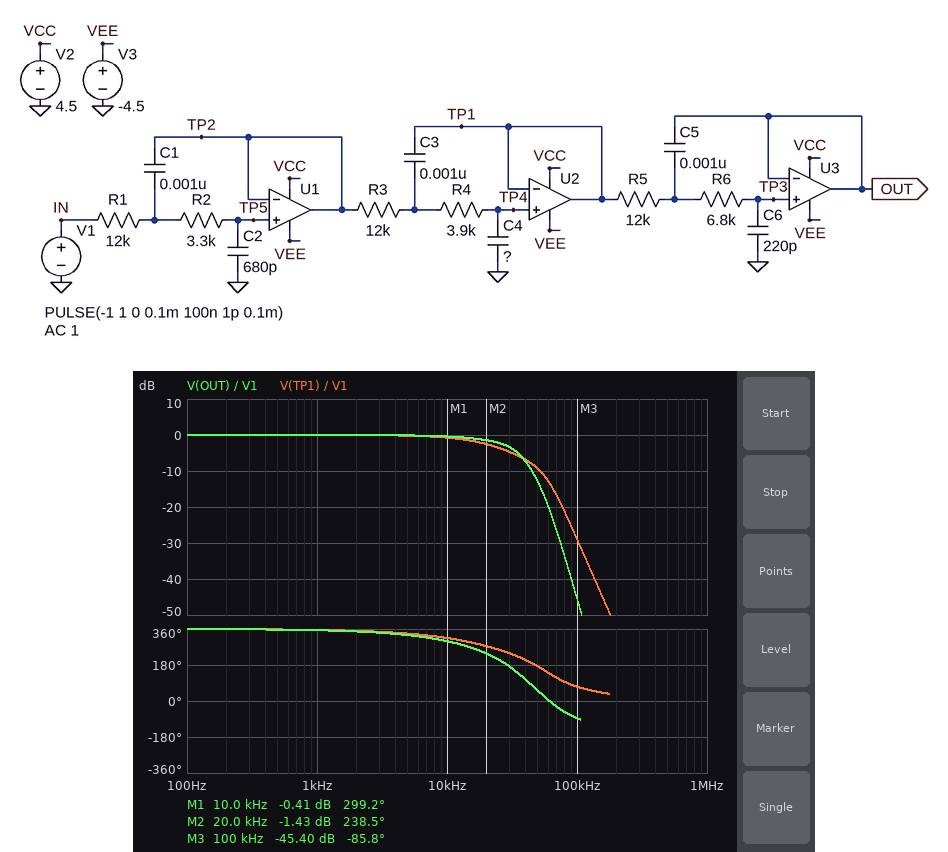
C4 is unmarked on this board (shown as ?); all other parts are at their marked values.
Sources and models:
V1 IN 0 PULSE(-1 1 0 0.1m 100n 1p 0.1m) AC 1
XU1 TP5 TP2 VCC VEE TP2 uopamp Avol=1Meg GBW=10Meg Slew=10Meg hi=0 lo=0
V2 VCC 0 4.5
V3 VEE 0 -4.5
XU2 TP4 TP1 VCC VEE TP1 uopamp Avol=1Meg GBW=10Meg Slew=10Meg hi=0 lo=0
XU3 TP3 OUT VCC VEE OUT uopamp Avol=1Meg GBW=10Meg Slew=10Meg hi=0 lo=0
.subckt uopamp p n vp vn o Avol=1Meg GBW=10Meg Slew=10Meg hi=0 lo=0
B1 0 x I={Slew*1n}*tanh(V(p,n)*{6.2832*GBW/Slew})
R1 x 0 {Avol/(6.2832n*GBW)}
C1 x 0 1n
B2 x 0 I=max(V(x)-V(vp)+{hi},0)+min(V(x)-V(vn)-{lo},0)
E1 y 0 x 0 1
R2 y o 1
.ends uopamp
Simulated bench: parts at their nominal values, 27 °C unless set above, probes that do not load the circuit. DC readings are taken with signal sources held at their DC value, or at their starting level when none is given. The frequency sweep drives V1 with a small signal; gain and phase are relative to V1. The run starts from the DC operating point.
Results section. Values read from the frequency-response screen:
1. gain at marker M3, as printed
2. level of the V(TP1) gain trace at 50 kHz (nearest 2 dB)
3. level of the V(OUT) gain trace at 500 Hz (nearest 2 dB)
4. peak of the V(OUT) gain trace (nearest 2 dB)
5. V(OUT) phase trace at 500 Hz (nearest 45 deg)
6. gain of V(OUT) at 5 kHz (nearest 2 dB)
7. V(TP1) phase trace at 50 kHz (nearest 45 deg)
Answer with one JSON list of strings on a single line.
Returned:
["-45.40 dB", "-10 dB", "0 dB", "0 dB", "360 deg", "0 dB", "180 deg"]
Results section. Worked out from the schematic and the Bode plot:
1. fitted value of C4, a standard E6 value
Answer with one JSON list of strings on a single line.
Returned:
["150 pF"]
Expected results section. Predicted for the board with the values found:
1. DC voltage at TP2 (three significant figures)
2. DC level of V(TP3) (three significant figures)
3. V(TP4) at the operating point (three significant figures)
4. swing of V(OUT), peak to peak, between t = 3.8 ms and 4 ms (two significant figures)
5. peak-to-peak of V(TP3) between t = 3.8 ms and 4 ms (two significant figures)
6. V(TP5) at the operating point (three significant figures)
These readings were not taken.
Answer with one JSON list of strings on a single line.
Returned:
["-1.00 V", "-1.00 V", "-1.00 V", "1.6 V", "1.6 V", "-1.00 V"]
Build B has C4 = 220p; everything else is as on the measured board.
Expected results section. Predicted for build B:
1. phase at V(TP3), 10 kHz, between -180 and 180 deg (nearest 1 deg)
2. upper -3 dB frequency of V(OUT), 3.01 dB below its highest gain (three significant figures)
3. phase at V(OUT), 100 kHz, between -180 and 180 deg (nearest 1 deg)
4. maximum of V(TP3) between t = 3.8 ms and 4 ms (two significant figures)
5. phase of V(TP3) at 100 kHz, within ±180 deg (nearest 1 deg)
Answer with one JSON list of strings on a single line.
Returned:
["-65 deg", "27.7 kHz", "-90 deg", "760 mV", "-89 deg"]
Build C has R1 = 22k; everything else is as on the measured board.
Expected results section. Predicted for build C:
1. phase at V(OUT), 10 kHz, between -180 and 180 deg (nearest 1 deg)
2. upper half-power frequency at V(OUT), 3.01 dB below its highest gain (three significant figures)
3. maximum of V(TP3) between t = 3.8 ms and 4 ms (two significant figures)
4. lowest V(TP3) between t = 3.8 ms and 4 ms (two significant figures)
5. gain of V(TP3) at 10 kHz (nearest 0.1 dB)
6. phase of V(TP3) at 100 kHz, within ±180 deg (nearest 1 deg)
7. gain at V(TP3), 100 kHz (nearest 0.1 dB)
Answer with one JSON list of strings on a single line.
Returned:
["-78 deg", "12.8 kHz", "650 mV", "-500 mV", "-2.1 dB", "-89 deg", "-50.7 dB"]
